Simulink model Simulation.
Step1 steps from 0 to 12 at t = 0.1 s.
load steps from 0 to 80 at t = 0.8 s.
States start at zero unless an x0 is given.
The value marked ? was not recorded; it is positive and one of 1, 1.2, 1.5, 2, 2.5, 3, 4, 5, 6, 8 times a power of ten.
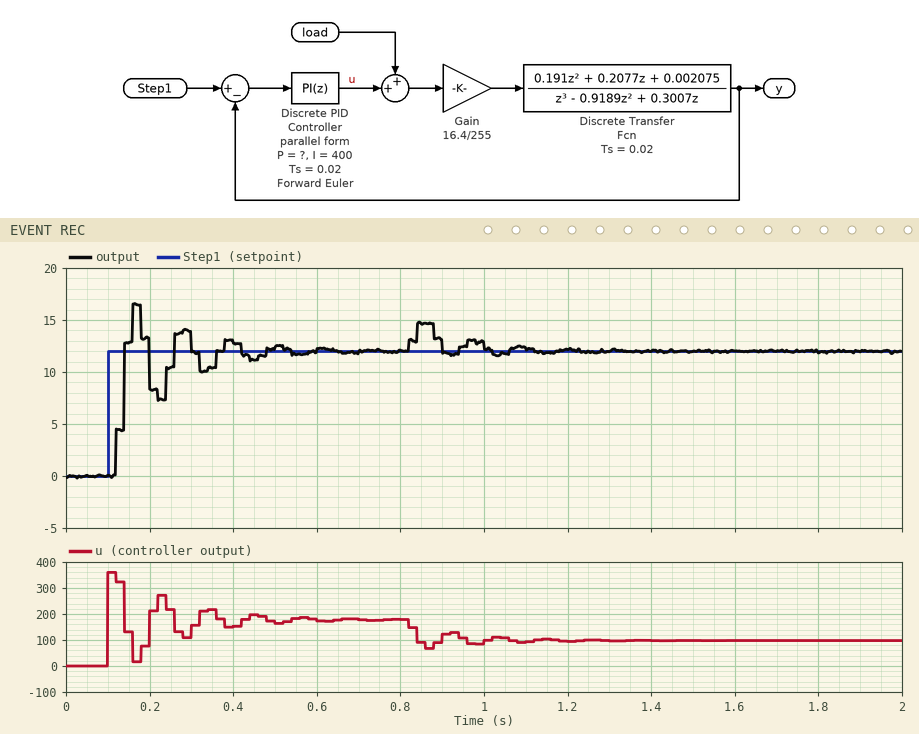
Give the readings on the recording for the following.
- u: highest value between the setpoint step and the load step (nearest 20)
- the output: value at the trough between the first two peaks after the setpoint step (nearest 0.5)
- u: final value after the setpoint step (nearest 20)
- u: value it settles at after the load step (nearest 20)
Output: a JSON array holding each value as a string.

["360", "7.5", "180", "100"]
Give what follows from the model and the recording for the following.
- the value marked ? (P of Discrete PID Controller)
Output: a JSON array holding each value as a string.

["30"]
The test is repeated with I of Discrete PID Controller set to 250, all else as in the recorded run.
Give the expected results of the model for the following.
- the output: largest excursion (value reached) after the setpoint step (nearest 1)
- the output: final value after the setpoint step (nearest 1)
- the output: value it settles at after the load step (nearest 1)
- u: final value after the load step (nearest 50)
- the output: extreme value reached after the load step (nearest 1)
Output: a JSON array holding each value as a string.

["15", "12", "12", "100", "15"]
